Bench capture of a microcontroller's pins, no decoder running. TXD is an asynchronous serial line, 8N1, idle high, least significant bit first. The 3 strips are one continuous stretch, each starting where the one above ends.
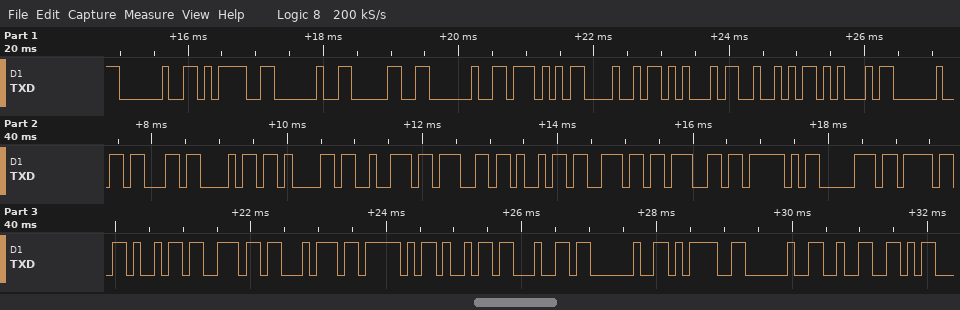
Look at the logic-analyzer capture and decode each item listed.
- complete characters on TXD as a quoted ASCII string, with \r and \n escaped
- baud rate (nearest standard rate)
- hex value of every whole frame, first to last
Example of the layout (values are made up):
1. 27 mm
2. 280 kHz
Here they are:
1. " = 0 WHERE charging_point_id = 2"
2. 9600 baud
3. 0x20 0x3D 0x20 0x30 0x20 0x57 0x48 0x45 0x52 0x45 0x20 0x63 0x68 0x61 0x72 0x67 0x69 0x6E 0x67 0x5F 0x70 0x6F 0x69 0x6E 0x74 0x5F 0x69 0x64 0x20 0x3D 0x20 0x32
